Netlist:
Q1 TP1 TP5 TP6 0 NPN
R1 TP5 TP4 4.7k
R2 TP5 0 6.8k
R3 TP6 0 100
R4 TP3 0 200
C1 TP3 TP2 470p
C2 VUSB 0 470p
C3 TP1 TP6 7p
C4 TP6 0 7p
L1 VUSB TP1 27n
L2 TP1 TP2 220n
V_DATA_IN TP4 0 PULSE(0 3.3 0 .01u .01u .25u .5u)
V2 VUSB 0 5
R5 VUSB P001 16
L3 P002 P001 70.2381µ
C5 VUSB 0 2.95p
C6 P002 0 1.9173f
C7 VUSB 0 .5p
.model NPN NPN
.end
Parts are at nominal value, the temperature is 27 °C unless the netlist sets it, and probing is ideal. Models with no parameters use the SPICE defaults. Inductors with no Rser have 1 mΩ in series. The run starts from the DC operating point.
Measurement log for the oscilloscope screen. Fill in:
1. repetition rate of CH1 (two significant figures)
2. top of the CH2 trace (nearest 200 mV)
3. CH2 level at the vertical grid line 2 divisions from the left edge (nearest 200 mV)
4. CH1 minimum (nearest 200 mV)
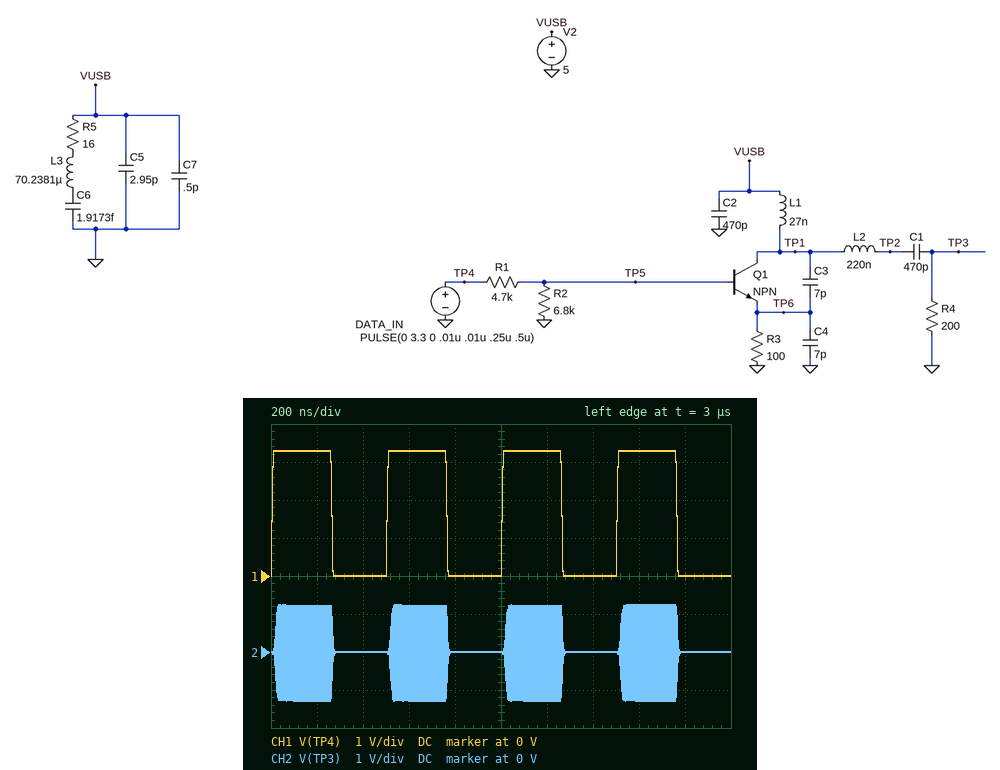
2.0 MHz
1.2 V
0 V
0 V
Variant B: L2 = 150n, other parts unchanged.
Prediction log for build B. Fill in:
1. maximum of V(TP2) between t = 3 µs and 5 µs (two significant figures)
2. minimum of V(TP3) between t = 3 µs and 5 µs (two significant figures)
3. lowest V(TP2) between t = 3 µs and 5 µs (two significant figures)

6.4 V
-1.5 V
3.5 V
